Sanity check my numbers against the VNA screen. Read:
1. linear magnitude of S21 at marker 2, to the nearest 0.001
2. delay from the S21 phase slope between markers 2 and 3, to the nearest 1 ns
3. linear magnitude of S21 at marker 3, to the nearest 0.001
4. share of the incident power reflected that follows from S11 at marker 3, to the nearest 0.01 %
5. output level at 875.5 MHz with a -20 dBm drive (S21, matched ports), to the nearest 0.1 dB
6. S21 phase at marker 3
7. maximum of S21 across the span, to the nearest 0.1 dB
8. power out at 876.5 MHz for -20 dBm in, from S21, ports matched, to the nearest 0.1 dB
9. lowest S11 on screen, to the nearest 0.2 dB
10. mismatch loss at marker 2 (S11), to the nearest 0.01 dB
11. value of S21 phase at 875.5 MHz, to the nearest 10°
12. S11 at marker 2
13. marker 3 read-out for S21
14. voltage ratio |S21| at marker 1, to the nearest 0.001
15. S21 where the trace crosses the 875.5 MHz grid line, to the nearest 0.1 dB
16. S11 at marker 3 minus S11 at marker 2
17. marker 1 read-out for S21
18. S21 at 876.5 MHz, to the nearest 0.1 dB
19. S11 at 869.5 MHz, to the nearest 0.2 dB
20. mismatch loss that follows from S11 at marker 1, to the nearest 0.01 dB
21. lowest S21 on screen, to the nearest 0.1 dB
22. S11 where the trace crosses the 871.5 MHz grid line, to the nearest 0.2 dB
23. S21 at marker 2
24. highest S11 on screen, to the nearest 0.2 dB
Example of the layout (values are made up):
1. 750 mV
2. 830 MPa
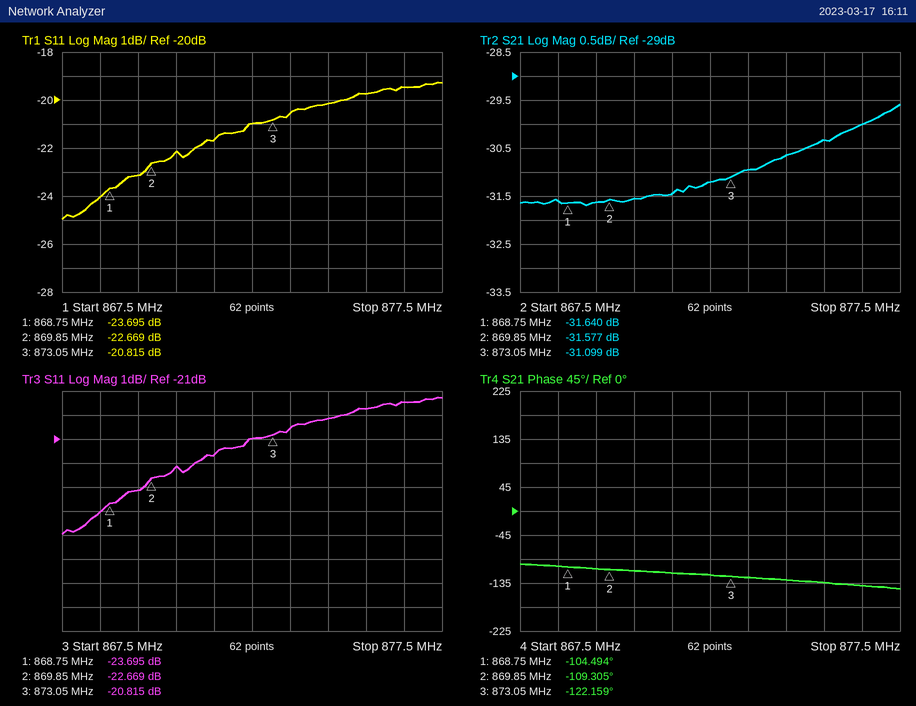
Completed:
1. 0.026
2. 11 ns
3. 0.028
4. 0.83 %
5. -50.3 dBm
6. -122.159°
7. -29.6 dB
8. -50.0 dBm
9. -25.0 dB
10. 0.02 dB
11. -130°
12. -22.669 dB
13. -31.099 dB
14. 0.026
15. -30.3 dB
16. 1.854 dB
17. -31.640 dB
18. -30.0 dB
19. -23.2 dB
20. 0.02 dB
21. -31.7 dB
22. -21.6 dB
23. -31.577 dB
24. -19.2 dB
